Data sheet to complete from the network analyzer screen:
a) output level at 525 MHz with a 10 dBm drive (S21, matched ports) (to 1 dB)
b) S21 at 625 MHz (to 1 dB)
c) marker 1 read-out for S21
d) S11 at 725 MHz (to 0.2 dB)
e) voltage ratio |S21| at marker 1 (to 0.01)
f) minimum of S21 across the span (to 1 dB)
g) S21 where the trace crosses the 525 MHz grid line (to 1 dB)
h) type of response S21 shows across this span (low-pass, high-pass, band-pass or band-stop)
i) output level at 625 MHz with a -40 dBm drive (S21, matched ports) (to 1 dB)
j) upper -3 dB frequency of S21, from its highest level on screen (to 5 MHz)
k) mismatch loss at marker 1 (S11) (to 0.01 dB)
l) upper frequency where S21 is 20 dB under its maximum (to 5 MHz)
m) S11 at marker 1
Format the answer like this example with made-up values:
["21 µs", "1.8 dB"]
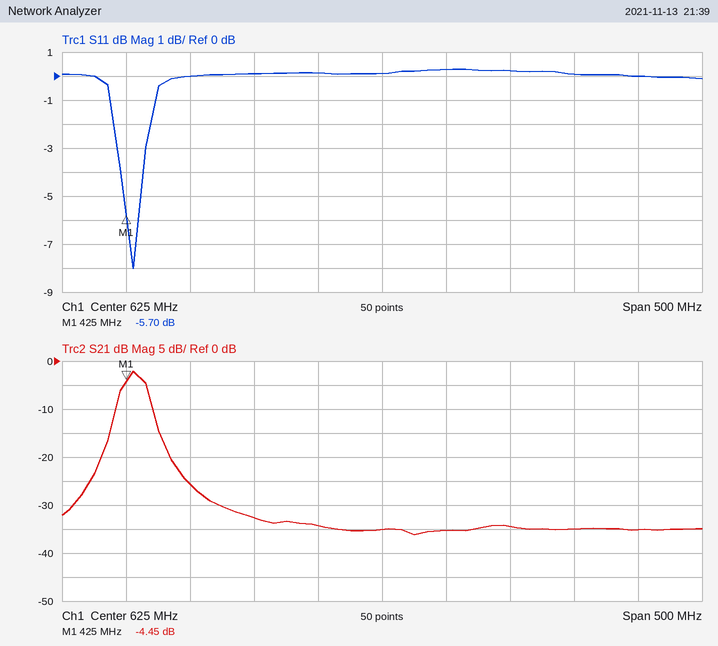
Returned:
["-23 dBm", "-35 dB", "-4.45 dB", "0.2 dB", "0.60", "-36 dB", "-33 dB", "band-pass", "-75 dBm", "440 MHz", "1.36 dB", "465 MHz", "-5.70 dB"]
